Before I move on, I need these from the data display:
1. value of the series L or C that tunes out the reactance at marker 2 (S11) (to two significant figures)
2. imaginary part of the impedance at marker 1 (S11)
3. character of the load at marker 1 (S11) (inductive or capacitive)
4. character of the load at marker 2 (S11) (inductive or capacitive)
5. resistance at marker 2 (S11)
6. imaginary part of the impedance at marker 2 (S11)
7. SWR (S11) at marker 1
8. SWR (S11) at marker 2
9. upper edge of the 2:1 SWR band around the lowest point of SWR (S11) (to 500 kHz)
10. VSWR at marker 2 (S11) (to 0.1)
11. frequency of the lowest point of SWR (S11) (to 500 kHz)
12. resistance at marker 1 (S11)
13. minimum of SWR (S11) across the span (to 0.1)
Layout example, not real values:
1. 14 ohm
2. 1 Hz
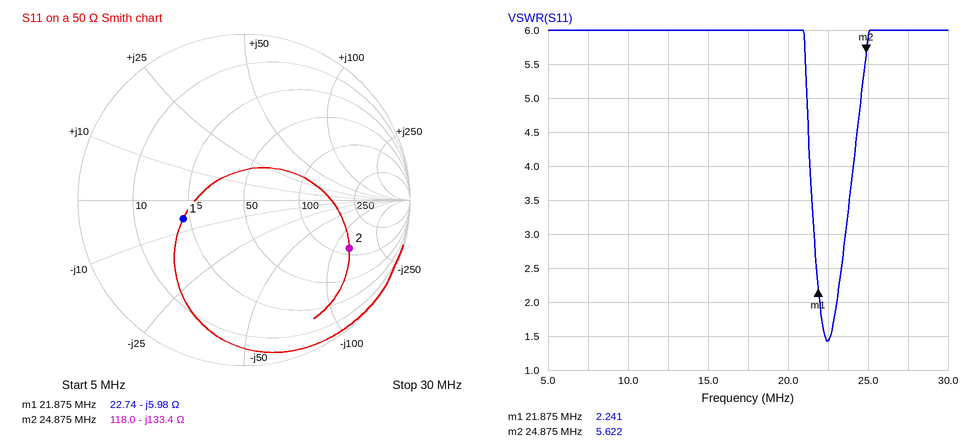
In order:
1. 850 nH
2. -5.98 Ω
3. capacitive
4. capacitive
5. 118.0 Ω
6. -133.4 Ω
7. 2.241
8. 5.622
9. 23.0 MHz
10. 5.6
11. 22.5 MHz
12. 22.74 Ω
13. 1.4
